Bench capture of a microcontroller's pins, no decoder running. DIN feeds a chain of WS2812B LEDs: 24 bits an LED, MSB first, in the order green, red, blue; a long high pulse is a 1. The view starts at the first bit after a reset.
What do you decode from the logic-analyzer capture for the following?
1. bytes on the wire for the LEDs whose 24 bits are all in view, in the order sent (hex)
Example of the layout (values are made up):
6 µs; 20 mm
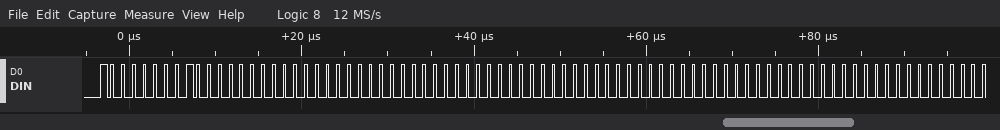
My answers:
80 80 00 00 00 00 00 00 00
